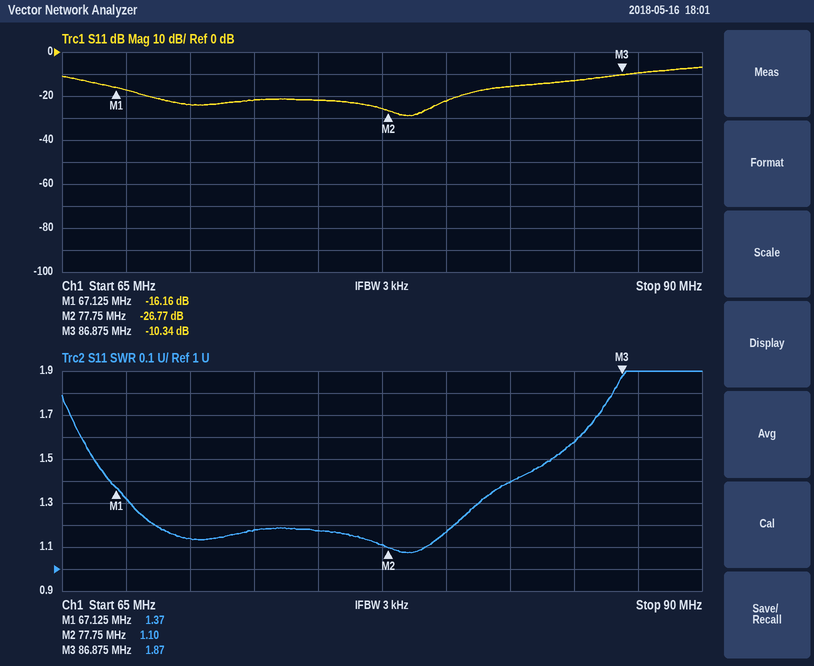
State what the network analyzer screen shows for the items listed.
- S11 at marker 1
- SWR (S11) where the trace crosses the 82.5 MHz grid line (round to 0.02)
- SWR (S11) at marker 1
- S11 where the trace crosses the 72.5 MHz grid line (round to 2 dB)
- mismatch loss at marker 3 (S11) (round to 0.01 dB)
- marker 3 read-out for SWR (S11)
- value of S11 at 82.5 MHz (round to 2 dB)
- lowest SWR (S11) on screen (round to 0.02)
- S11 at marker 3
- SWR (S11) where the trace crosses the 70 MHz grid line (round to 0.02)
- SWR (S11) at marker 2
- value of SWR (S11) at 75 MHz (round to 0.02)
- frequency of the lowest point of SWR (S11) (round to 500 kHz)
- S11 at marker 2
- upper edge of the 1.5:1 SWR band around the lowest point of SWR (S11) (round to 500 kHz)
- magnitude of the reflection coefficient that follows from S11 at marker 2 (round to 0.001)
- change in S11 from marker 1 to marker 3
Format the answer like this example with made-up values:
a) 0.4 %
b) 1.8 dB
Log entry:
a) -16.16 dB
b) 1.40
c) 1.37
d) -22 dB
e) 0.42 dB
f) 1.87
g) -16 dB
h) 1.08
i) -10.34 dB
j) 1.14
k) 1.10
l) 1.18
m) 78.5 MHz
n) -26.77 dB
o) 84.0 MHz
p) 0.046
q) 5.82 dB
